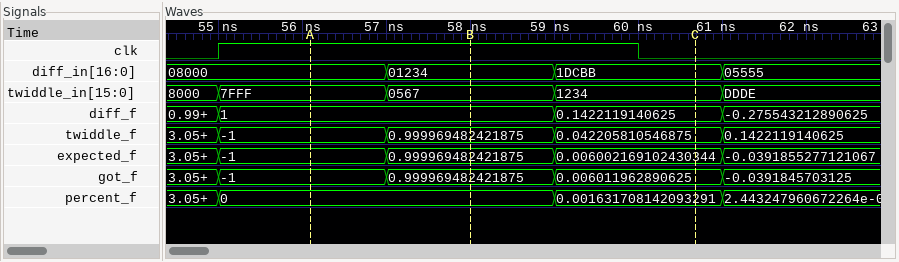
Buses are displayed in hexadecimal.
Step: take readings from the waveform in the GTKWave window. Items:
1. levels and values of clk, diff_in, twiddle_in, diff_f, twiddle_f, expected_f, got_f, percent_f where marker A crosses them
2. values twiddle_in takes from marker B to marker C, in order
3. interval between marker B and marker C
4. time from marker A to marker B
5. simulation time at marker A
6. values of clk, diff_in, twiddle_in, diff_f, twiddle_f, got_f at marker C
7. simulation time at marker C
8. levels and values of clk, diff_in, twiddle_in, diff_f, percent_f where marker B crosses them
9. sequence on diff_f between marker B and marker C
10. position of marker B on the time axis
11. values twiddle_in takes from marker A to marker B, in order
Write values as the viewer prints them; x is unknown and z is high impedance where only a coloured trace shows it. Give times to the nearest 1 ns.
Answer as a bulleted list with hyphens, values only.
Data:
- clk=1, diff_in=08000, twiddle_in=7FFF, diff_f=1, twiddle_f=-1, expected_f=-1, got_f=-1, percent_f=0
- 0567, 1234
- 3 ns
- 2 ns
- 56 ns
- clk=0, diff_in=1DCBB, twiddle_in=1234, diff_f=0.1422119140625, twiddle_f=0.042205810546875, got_f=0.006011962890625
- 61 ns
- clk=1, diff_in=01234, twiddle_in=0567, diff_f=1, percent_f=0
- 1, 0.1422119140625
- 58 ns
- 7FFF, 0567
